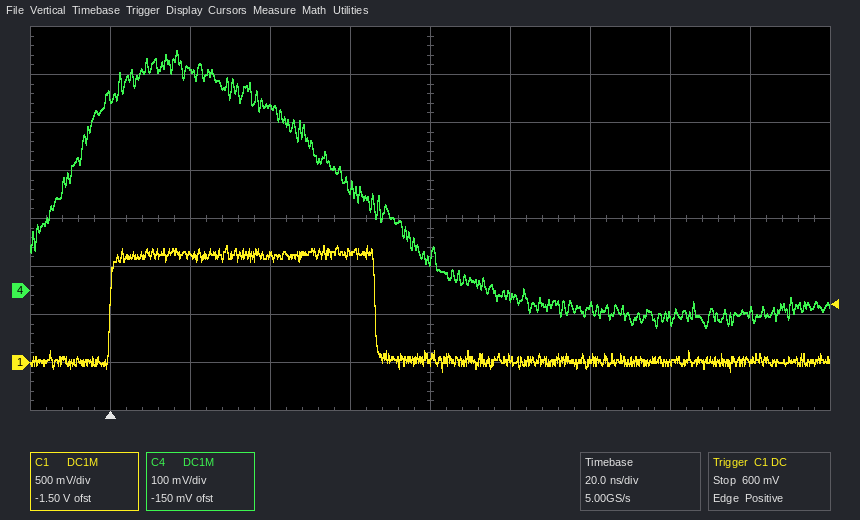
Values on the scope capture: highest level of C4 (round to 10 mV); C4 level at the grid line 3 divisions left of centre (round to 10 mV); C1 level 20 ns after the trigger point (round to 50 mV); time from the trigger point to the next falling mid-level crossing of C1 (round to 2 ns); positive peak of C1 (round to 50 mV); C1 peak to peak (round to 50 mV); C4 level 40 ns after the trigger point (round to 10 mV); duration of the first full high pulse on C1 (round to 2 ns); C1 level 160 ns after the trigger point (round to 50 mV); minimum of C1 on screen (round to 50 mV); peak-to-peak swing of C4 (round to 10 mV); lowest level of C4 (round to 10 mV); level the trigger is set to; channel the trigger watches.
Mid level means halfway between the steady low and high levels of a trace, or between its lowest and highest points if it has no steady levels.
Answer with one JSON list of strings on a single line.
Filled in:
["500 mV", "460 mV", "1.10 V", "66 ns", "1.20 V", "1.30 V", "380 mV", "66 ns", "0 mV", "-100 mV", "580 mV", "-80 mV", "600 mV", "C1"]
